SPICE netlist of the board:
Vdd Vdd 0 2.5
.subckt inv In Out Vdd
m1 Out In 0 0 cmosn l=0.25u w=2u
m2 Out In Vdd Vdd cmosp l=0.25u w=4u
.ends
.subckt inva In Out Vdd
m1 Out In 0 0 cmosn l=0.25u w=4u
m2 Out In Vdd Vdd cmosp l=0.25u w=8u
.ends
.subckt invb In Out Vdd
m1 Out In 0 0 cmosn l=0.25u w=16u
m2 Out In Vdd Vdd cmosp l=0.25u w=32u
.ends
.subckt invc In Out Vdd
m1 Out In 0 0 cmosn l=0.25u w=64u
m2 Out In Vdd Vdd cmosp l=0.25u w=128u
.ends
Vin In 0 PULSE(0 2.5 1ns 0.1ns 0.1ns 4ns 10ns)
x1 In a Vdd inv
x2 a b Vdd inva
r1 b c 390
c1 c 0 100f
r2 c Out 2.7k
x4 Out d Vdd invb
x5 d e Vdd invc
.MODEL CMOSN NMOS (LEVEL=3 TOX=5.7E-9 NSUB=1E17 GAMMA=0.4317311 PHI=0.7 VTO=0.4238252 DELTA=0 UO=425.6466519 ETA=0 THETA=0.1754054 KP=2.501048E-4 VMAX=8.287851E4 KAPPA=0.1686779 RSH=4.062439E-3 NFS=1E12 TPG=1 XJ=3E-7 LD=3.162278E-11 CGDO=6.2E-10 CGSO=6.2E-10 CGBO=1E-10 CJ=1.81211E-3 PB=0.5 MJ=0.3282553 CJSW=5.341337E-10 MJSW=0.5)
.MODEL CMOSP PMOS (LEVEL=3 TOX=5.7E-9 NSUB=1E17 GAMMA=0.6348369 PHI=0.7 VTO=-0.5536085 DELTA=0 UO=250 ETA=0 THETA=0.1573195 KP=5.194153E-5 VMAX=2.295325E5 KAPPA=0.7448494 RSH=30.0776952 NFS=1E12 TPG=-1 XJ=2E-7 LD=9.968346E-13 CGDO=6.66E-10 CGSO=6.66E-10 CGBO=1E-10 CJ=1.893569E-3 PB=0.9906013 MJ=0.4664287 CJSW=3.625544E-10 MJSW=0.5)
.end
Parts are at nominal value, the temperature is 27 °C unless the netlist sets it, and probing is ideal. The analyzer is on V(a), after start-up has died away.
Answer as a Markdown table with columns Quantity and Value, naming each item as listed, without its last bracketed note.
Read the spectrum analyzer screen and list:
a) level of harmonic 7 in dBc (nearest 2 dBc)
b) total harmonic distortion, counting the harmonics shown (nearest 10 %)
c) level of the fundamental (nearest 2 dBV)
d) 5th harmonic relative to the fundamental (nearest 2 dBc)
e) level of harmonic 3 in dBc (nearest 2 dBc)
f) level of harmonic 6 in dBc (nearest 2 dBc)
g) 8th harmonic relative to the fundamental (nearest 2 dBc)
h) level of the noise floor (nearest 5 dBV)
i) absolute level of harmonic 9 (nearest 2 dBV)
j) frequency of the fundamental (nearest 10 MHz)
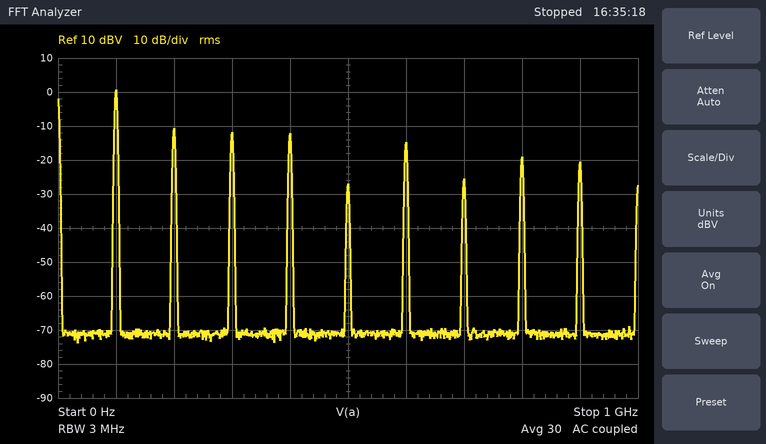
| Quantity | Value |
|---|---|
| level of harmonic 7 in dBc | -26 dBc |
| total harmonic distortion, counting the harmonics shown | 50 % |
| level of the fundamental | 0 dBV |
| 5th harmonic relative to the fundamental | -28 dBc |
| level of harmonic 3 in dBc | -12 dBc |
| level of harmonic 6 in dBc | -16 dBc |
| 8th harmonic relative to the fundamental | -20 dBc |
| level of the noise floor | -70 dBV |
| absolute level of harmonic 9 | -20 dBV |
| frequency of the fundamental | 100 MHz |
